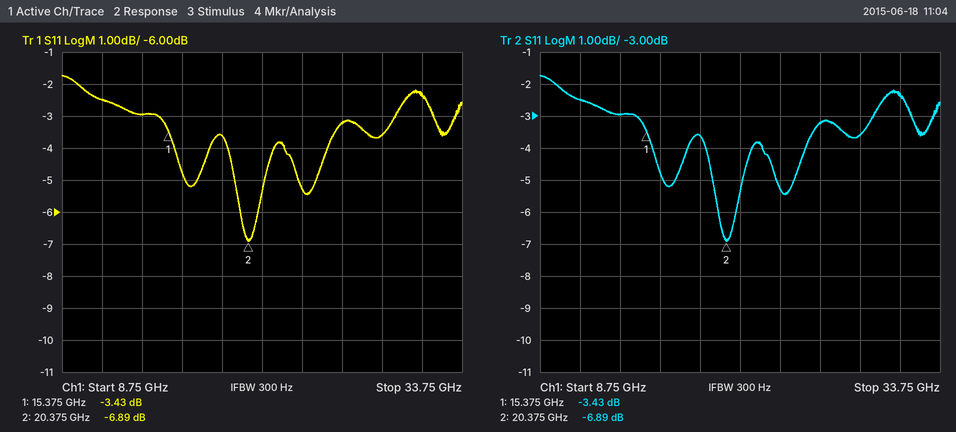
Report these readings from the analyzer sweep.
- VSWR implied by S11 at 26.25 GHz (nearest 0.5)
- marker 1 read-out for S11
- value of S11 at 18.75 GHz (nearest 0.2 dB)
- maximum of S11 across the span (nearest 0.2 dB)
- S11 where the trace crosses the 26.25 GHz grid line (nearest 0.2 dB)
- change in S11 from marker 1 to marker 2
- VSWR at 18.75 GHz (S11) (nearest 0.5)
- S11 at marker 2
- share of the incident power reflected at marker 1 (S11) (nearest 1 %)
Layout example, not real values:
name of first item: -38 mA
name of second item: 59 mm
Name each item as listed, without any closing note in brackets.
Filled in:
VSWR implied by S11 at 26.25 GHz: 5.5
marker 1 read-out for S11: -3.43 dB
value of S11 at 18.75 GHz: -3.6 dB
maximum of S11 across the span: -1.8 dB
S11 where the trace crosses the 26.25 GHz grid line: -3.2 dB
change in S11 from marker 1 to marker 2: -3.46 dB
VSWR at 18.75 GHz (S11): 5.0
S11 at marker 2: -6.89 dB
share of the incident power reflected at marker 1 (S11): 45 %
